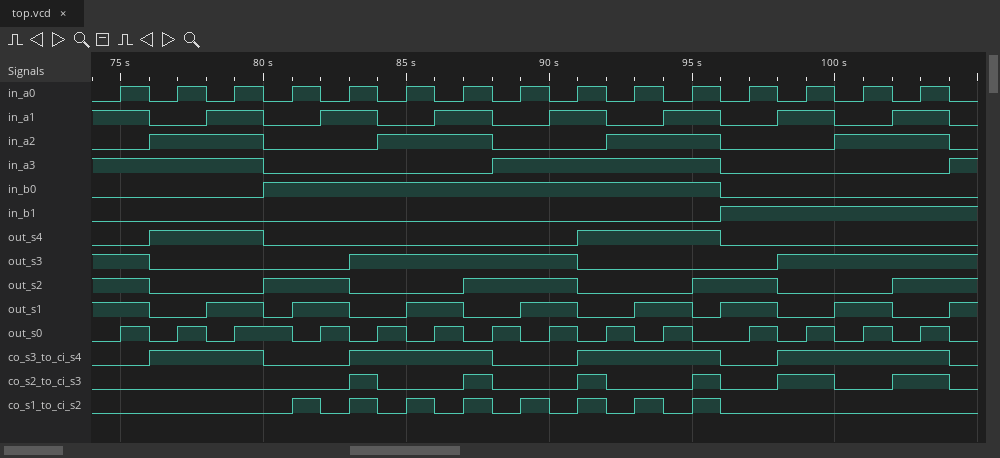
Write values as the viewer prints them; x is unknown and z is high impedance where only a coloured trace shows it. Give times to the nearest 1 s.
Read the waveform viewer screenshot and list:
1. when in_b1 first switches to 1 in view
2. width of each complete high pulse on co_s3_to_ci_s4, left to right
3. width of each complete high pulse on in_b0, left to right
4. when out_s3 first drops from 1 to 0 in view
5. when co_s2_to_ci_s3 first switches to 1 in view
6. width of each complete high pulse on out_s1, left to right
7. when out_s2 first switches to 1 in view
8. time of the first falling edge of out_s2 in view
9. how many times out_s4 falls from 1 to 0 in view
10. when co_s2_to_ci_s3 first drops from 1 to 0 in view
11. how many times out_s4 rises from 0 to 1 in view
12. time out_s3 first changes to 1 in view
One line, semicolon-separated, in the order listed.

96 s; 4 s, 5 s, 5 s, 6 s; 16 s; 76 s; 83 s; 2 s, 2 s, 2 s, 2 s, 2 s, 2 s, 2 s; 80 s; 76 s; 2; 84 s; 2; 83 s
